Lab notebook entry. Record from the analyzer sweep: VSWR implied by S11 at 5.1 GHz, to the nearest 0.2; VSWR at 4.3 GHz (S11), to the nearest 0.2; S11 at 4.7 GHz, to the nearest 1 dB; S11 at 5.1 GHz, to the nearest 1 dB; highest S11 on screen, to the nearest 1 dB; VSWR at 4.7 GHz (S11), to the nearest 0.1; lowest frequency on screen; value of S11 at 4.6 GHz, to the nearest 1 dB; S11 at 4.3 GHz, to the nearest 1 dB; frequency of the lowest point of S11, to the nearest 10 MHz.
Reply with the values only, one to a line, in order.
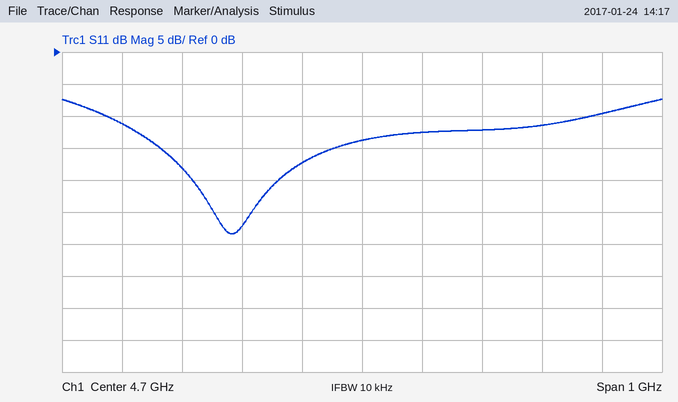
2.0
1.8
-14 dB
-10 dB
-7 dB
1.5
4.2 GHz
-17 dB
-11 dB
4.48 GHz
